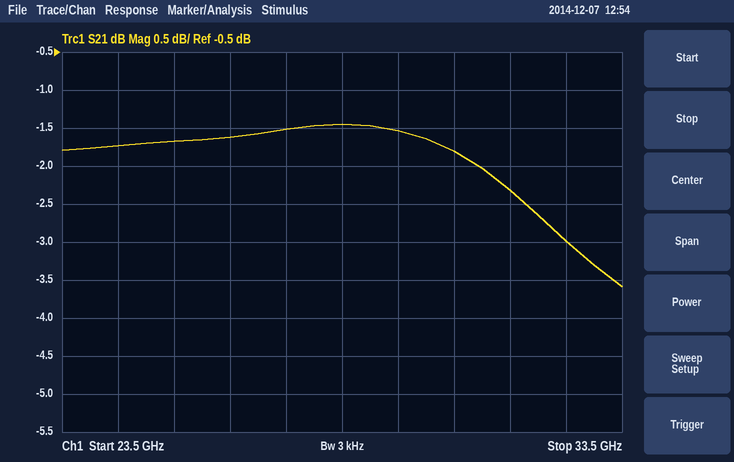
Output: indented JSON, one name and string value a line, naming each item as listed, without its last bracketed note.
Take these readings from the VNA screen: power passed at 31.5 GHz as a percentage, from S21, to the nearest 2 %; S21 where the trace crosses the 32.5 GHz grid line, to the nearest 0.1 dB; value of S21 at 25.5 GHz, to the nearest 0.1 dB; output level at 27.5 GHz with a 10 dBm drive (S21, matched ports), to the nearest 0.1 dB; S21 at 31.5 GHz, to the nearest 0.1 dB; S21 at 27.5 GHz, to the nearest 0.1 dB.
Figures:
{
  "power passed at 31.5 GHz as a percentage, from S21, to the nearest 2 %": "58 %",
  "S21 where the trace crosses the 32.5 GHz grid line, to the nearest 0.1 dB": "-3.0 dB",
  "value of S21 at 25.5 GHz, to the nearest 0.1 dB": "-1.7 dB",
  "output level at 27.5 GHz with a 10 dBm drive (S21, matched ports), to the nearest 0.1 dB": "8.5 dBm",
  "S21 at 31.5 GHz, to the nearest 0.1 dB": "-2.3 dB",
  "S21 at 27.5 GHz, to the nearest 0.1 dB": "-1.5 dB"
}
